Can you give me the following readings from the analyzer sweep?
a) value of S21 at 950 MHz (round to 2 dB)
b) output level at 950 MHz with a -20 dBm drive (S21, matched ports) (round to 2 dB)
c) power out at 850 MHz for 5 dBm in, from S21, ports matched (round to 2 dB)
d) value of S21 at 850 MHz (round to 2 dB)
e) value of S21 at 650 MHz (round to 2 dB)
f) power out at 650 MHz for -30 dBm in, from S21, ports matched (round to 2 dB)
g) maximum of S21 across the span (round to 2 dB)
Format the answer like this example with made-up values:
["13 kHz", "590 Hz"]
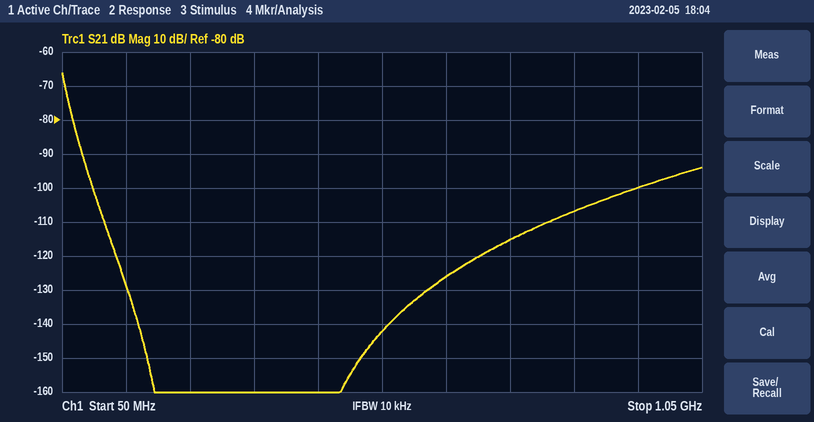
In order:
["-100 dB", "-120 dBm", "-102 dBm", "-106 dB", "-126 dB", "-156 dBm", "-66 dB"]
